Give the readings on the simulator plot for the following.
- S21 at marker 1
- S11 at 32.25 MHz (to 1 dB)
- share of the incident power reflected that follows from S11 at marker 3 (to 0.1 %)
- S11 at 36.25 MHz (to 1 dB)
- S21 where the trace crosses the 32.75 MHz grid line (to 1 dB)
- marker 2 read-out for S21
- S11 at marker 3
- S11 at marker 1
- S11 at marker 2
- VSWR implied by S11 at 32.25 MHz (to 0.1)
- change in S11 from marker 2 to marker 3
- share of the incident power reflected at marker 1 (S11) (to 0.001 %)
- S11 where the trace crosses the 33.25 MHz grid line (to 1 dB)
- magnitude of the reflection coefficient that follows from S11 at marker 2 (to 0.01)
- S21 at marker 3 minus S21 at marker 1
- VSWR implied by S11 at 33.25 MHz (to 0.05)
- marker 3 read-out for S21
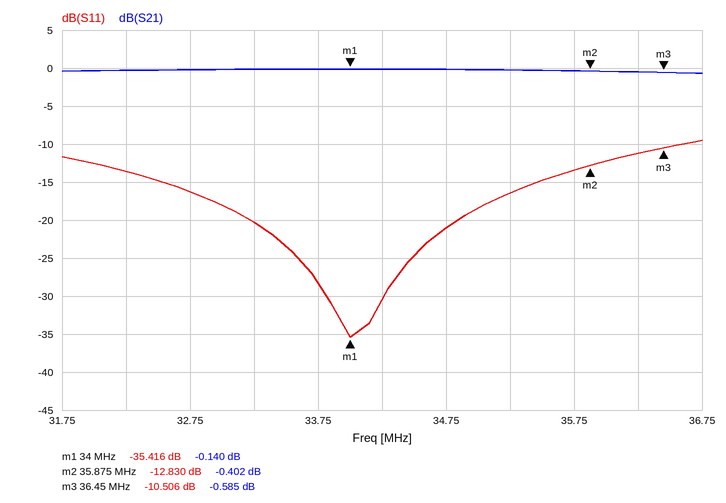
-0.140 dB
-14 dB
8.9 %
-11 dB
0 dB
-0.402 dB
-10.506 dB
-35.416 dB
-12.830 dB
1.5
2.324 dB
0.029 %
-20 dB
0.23
-0.445 dB
1.20
-0.585 dB
